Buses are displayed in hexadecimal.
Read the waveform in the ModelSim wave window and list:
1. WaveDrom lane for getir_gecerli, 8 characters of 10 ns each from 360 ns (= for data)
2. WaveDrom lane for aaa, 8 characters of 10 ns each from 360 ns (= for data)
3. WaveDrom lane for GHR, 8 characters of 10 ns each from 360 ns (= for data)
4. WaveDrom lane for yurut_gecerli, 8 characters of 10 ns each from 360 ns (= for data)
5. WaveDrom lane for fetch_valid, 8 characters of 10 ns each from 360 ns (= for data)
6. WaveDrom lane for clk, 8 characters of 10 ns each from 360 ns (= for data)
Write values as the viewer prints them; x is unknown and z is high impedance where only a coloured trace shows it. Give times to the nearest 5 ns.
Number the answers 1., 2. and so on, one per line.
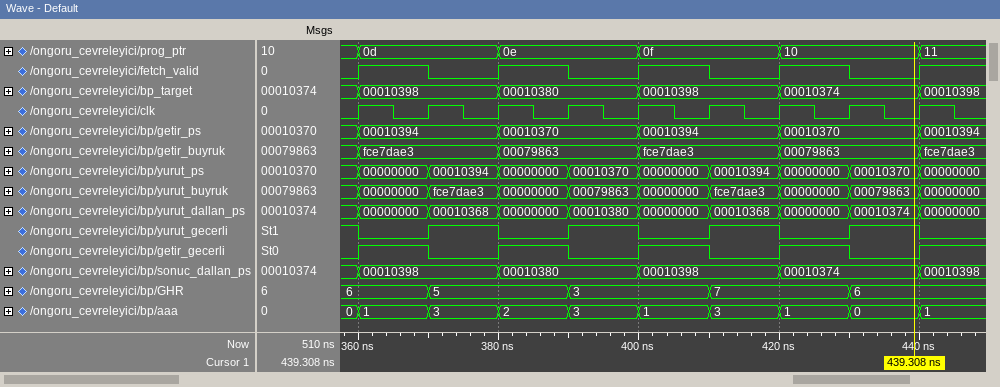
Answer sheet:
1. {name: 'getir_gecerli', wave: '10101010'}
2. {name: 'aaa', wave: '========', data: '1 3 2 3 1 3 1 0'}
3. {name: 'GHR', wave: '==.=.=.=', data: '6 5 3 7 6'}
4. {name: 'yurut_gecerli', wave: '01010101'}
5. {name: 'fetch_valid', wave: '10101010'}
6. {name: 'clk', wave: 'p.......'}
